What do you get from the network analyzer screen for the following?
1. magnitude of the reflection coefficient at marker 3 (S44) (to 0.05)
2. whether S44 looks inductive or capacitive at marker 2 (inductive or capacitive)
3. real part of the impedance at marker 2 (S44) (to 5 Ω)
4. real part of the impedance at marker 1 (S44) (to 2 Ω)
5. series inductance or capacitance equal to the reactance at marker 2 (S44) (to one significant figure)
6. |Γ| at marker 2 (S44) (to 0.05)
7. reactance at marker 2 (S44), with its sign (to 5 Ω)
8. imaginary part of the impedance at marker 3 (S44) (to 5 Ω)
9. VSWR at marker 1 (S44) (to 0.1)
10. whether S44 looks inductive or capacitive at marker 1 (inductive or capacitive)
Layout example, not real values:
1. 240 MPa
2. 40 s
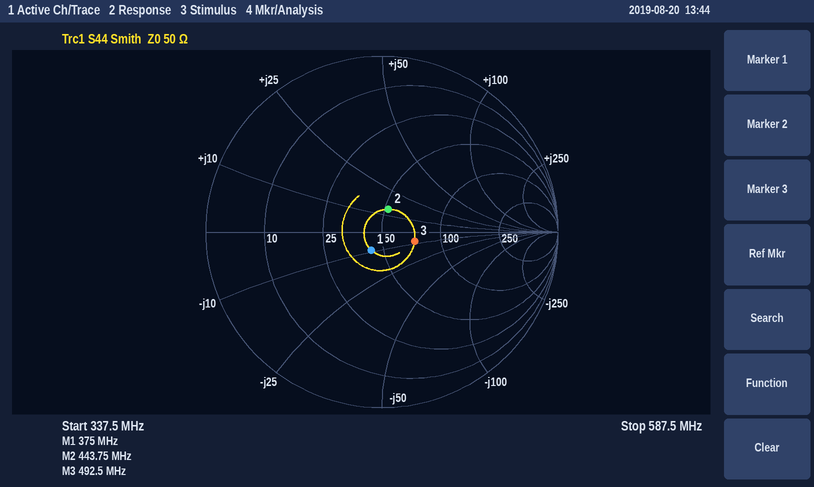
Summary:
1. 0.20
2. inductive
3. 50 Ω
4. 44 Ω
5. 5 nH
6. 0.15
7. +15 Ω
8. -10 Ω
9. 1.3
10. capacitive
